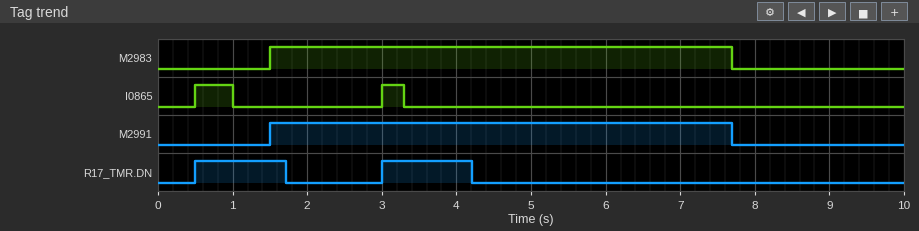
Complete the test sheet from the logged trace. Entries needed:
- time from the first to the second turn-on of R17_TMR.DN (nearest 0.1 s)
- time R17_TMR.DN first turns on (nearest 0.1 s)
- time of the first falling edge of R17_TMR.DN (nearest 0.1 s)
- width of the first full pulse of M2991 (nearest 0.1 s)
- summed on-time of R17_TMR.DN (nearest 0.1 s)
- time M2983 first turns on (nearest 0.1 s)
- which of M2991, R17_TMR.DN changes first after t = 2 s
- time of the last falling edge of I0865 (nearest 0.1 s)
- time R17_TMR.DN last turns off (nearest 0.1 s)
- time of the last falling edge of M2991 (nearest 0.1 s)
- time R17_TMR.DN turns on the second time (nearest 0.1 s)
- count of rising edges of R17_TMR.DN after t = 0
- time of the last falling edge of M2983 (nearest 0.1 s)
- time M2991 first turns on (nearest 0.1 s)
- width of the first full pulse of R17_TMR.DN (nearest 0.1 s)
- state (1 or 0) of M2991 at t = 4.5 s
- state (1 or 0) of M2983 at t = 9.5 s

2.5 s
0.5 s
1.7 s
6.2 s
2.4 s
1.5 s
R17_TMR.DN
3.3 s
4.2 s
7.7 s
3.0 s
2
7.7 s
1.5 s
1.2 s
1
0
